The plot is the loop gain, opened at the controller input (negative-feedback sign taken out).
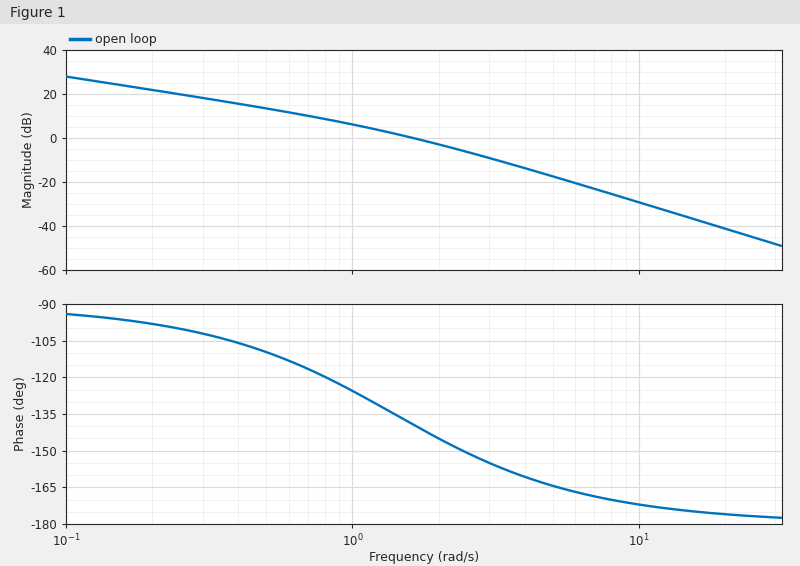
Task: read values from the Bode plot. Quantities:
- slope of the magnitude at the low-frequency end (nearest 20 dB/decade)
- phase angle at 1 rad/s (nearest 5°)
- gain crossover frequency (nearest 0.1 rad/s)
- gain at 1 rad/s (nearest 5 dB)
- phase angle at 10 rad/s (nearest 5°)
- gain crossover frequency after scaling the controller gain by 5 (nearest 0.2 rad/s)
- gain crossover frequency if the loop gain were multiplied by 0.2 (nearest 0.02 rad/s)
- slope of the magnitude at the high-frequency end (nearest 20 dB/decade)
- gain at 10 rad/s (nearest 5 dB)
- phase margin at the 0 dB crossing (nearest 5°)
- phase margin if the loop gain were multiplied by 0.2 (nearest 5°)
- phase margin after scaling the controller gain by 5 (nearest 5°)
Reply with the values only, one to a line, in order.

-20 dB/decade
-125°
1.6 rad/s
5 dB
-170°
4.0 rad/s
0.48 rad/s
-40 dB/decade
-30 dB
40°
70°
20°
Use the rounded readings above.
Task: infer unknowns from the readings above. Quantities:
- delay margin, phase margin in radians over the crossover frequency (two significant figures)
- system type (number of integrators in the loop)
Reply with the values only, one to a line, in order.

0.44 s
1
